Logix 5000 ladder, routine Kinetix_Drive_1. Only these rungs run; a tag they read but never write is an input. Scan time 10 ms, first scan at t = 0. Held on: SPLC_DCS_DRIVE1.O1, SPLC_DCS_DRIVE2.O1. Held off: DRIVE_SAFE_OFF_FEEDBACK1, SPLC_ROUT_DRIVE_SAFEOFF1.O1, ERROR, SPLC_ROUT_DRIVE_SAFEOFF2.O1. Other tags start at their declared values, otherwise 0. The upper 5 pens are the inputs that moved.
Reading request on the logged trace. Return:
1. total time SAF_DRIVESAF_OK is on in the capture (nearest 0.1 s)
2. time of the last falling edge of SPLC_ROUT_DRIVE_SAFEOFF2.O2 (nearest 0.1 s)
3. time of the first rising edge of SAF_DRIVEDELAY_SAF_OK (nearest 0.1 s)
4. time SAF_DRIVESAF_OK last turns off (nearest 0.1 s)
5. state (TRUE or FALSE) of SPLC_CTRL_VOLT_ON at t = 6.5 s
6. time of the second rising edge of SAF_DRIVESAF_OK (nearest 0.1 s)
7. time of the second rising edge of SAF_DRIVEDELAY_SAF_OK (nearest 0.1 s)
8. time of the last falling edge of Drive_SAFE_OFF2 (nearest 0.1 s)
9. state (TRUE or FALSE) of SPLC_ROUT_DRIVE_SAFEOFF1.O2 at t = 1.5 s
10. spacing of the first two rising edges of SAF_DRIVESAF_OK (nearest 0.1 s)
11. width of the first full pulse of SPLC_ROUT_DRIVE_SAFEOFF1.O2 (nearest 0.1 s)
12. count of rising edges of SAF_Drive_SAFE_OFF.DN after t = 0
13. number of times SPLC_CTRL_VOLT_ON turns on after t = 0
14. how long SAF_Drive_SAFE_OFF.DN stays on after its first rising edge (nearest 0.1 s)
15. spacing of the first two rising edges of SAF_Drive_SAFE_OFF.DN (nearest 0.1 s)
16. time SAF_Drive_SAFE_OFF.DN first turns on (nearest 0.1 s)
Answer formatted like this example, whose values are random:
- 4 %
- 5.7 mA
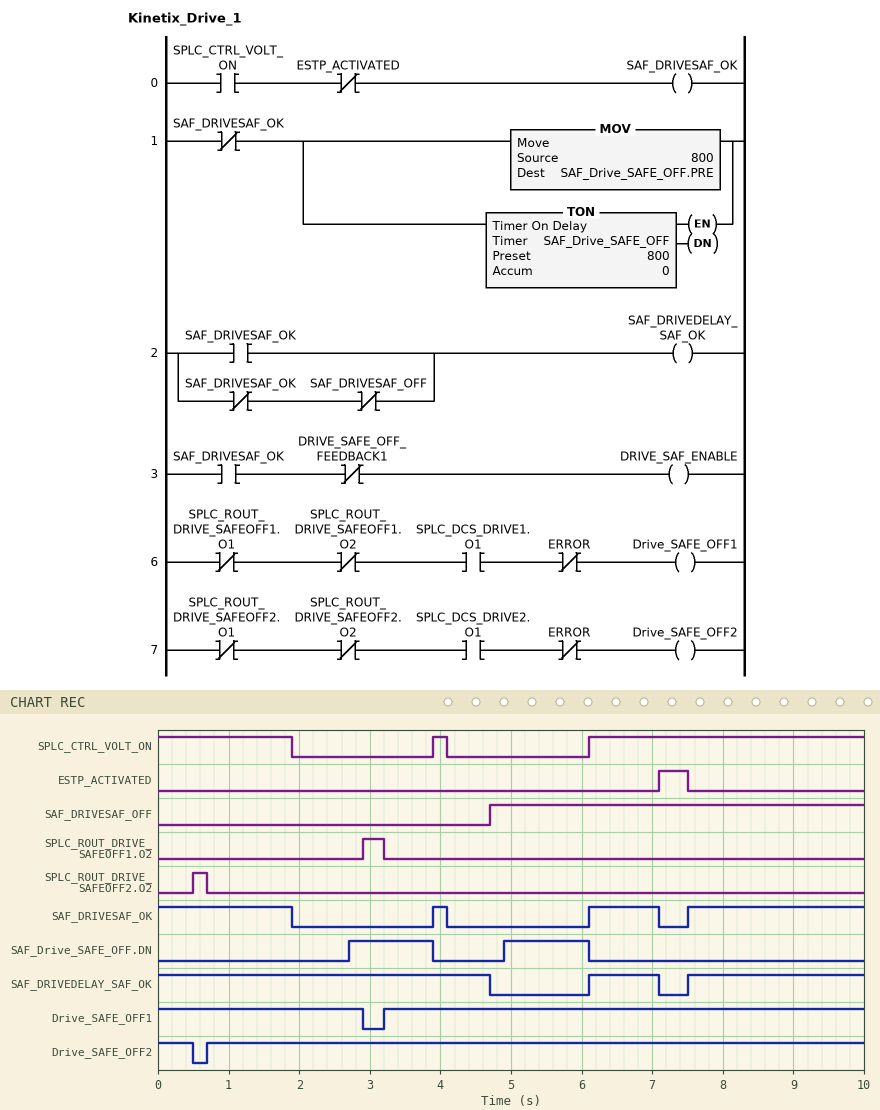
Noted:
- 5.6 s
- 0.7 s
- 6.1 s
- 7.1 s
- TRUE
- 6.1 s
- 7.5 s
- 0.5 s
- FALSE
- 2.2 s
- 0.3 s
- 2
- 2
- 1.2 s
- 2.2 s
- 2.7 s
